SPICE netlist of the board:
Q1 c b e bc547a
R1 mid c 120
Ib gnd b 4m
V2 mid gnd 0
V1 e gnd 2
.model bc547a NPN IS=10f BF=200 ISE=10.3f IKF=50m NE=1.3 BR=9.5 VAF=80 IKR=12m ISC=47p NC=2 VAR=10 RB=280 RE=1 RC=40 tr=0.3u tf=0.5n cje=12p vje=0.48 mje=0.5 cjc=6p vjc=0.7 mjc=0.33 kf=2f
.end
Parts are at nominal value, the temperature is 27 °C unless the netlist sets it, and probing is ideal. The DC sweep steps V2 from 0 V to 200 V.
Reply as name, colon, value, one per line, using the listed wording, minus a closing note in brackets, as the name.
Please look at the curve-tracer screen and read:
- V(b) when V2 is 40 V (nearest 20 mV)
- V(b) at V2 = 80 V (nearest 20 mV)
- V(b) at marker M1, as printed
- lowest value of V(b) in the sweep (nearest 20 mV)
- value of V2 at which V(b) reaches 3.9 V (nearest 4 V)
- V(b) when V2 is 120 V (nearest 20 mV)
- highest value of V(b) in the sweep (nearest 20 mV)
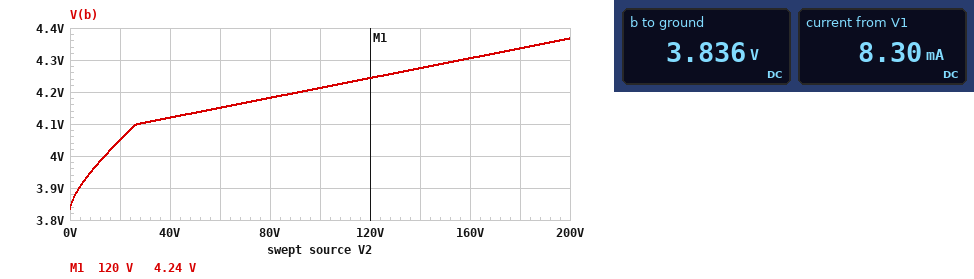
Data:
V(b) when V2 is 40 V: 4.12 V
V(b) at V2 = 80 V: 4.18 V
V(b) at marker M1, as printed: 4.24 V
lowest value of V(b) in the sweep: 3.84 V
value of V2 at which V(b) reaches 3.9 V: 4 V
V(b) when V2 is 120 V: 4.24 V
highest value of V(b) in the sweep: 4.36 V
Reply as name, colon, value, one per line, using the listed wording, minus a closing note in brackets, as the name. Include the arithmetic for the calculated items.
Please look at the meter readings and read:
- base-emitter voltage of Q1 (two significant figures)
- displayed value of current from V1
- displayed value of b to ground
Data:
base-emitter voltage of Q1: 3.836 V - 2 V = 1.8 V
displayed value of current from V1: 8.30 mA
displayed value of b to ground: 3.836 V
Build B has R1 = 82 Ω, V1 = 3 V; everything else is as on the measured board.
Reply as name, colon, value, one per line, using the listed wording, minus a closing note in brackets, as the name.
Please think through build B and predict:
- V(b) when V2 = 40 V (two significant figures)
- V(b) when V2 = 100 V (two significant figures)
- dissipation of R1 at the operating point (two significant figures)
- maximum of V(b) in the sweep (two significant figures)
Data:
V(b) when V2 = 40 V: 5.1 V
V(b) when V2 = 100 V: 5.2 V
dissipation of R1 at the operating point: 31 mW
maximum of V(b) in the sweep: 5.4 V
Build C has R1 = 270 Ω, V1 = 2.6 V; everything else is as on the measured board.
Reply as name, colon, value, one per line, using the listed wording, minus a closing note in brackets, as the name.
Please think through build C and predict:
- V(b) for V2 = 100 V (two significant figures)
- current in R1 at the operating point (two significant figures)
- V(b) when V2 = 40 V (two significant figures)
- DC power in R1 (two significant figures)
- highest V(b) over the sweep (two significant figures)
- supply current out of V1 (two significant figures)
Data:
V(b) for V2 = 100 V: 4.8 V
current in R1 at the operating point: 8.3 mA
V(b) when V2 = 40 V: 4.7 V
DC power in R1: 19 mW
highest V(b) over the sweep: 4.9 V
supply current out of V1: 4.3 mA
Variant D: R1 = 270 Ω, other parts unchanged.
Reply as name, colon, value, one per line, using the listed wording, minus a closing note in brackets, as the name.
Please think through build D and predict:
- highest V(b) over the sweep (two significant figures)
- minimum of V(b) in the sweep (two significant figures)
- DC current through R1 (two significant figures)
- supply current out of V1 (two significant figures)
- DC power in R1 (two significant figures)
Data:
highest V(b) over the sweep: 4.3 V
minimum of V(b) in the sweep: 3.9 V
DC current through R1: 6.4 mA
supply current out of V1: 2.4 mA
DC power in R1: 11 mW
